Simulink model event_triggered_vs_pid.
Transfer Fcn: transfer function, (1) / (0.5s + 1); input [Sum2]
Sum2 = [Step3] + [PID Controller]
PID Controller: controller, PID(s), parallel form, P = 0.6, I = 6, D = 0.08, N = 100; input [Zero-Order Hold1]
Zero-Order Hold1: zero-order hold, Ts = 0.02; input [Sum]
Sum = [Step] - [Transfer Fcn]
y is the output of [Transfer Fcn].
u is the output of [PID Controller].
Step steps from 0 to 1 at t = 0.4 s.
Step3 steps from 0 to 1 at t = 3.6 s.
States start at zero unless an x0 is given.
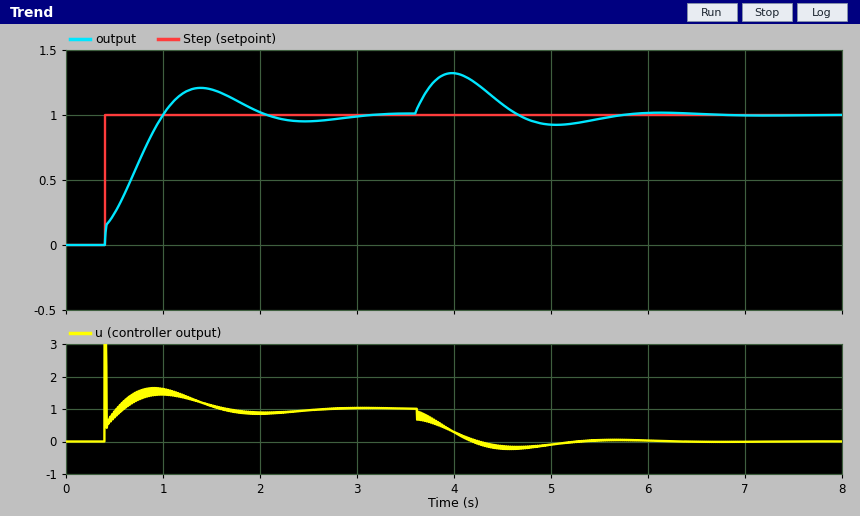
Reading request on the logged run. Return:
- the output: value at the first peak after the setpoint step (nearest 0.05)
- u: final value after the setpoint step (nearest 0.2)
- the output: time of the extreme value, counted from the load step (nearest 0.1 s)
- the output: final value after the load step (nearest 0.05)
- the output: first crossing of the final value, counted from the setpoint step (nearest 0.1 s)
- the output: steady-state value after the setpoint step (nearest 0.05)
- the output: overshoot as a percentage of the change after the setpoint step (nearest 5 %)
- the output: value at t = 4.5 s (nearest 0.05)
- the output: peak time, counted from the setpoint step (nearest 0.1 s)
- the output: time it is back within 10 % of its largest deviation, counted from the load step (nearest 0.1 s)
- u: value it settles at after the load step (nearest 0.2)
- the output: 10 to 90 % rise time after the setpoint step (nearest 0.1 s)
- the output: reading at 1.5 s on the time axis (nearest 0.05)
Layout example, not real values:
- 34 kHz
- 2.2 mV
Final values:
- 1.20
- 1.0
- 0.4 s
- 1.00
- 0.6 s
- 1.00
- 20 %
- 1.10
- 1.0 s
- 1.9 s
- 0.0
- 0.5 s
- 1.20
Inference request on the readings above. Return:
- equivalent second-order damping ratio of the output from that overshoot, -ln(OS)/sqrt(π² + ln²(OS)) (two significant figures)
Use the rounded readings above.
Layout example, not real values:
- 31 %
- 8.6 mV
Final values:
- 0.46
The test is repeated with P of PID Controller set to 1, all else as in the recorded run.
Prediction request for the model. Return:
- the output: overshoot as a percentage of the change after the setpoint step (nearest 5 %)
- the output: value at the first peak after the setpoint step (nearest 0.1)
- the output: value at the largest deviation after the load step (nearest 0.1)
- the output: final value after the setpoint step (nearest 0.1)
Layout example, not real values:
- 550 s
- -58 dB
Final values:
- 15 %
- 1.1
- 1.3
- 1.0
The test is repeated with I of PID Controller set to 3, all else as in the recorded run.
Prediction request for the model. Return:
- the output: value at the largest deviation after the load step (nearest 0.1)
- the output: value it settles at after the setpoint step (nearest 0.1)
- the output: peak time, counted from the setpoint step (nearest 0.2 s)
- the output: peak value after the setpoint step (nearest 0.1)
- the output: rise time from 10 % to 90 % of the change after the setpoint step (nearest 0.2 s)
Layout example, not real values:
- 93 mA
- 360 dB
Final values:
- 1.4
- 1.0
- 1.6 s
- 1.1
- 0.8 s
